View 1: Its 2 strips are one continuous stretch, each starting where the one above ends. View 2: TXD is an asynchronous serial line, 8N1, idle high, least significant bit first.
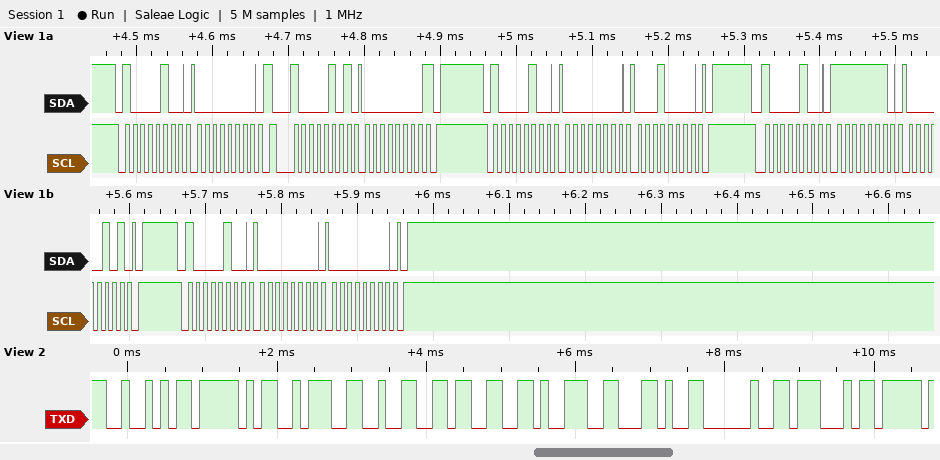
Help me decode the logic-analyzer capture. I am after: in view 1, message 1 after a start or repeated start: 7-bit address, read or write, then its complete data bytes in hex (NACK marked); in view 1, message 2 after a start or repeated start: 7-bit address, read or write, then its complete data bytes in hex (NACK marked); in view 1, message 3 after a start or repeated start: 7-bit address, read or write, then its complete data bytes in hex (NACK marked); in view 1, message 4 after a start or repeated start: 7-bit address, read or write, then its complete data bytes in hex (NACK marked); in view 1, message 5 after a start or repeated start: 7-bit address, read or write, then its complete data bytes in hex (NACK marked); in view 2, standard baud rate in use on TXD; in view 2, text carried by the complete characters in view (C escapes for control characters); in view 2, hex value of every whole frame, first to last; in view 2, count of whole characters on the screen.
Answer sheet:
0x42 write: 00
0x42 read: 00 NACK
0x42 write: 00 10
0x42 write: FE 05
0x42 write: 00 00
9600 baud
"R_:239, G"
52 5F 3A 32 33 39 2C 20 47
9
